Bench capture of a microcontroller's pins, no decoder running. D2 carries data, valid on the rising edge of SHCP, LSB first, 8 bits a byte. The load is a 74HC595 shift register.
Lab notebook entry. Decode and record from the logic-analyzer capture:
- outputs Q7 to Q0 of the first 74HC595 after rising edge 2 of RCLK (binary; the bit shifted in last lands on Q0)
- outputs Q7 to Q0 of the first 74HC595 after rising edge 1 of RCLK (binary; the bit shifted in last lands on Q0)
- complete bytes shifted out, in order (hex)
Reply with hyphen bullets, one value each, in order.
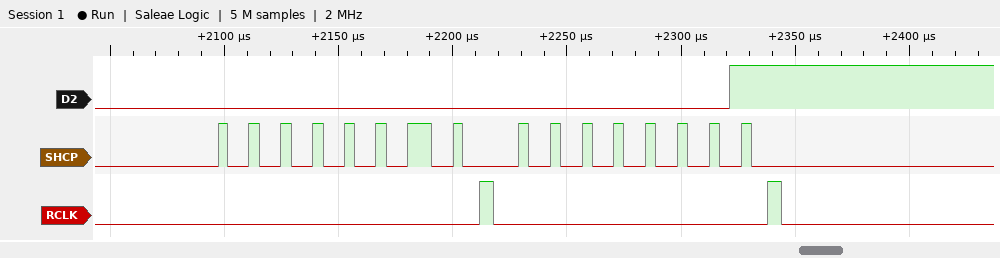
- 00000001
- 00000000
- 0x00 0x80
